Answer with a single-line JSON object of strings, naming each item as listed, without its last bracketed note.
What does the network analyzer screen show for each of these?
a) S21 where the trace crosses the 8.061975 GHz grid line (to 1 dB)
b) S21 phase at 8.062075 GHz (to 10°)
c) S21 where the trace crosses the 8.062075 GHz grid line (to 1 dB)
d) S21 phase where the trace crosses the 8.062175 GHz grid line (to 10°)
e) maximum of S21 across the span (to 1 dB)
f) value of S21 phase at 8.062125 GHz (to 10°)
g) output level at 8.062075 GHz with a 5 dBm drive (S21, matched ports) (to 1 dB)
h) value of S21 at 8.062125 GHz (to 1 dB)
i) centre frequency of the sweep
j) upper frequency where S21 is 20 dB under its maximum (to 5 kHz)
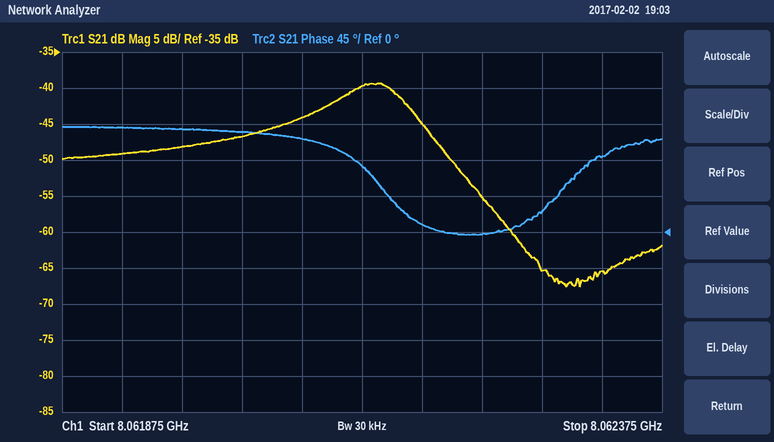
{"S21 where the trace crosses the 8.061975 GHz grid line": "-48 dB", "S21 phase at 8.062075 GHz": "120°", "S21 where the trace crosses the 8.062075 GHz grid line": "-44 dB", "S21 phase where the trace crosses the 8.062175 GHz grid line": "10°", "maximum of S21 across the span": "-39 dB", "value of S21 phase at 8.062125 GHz": "80°", "output level at 8.062075 GHz with a 5 dBm drive (S21, matched ports)": "-39 dBm", "value of S21 at 8.062125 GHz": "-40 dB", "centre frequency of the sweep": "8.062125 GHz", "upper frequency where S21 is 20 dB under its maximum": "8.062245 GHz"}
